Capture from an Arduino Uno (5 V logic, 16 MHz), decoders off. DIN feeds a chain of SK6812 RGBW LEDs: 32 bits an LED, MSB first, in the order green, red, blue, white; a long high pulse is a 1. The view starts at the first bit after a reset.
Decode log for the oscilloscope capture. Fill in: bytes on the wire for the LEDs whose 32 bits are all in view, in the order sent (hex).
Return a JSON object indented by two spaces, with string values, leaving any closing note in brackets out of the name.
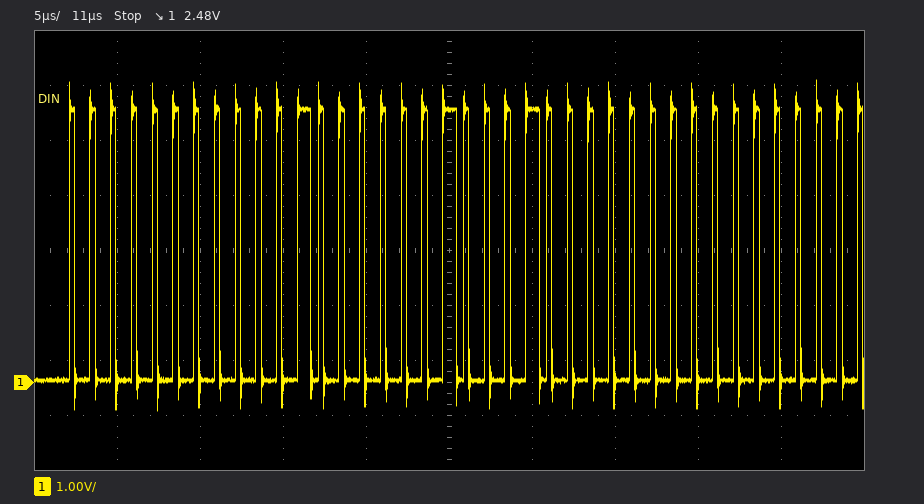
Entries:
{
  "bytes on the wire for the LEDs whose 32 bits are all in view, in the order sent": "00 10 22 00"
}
